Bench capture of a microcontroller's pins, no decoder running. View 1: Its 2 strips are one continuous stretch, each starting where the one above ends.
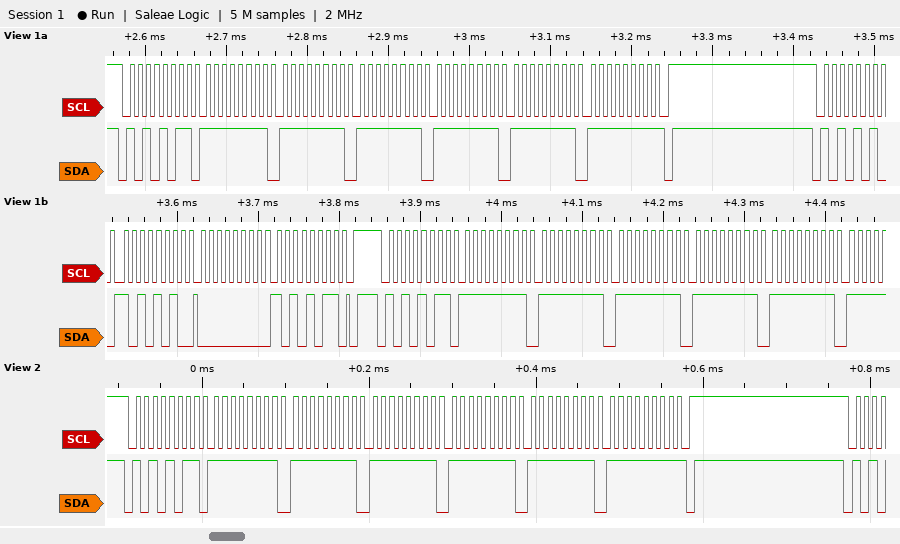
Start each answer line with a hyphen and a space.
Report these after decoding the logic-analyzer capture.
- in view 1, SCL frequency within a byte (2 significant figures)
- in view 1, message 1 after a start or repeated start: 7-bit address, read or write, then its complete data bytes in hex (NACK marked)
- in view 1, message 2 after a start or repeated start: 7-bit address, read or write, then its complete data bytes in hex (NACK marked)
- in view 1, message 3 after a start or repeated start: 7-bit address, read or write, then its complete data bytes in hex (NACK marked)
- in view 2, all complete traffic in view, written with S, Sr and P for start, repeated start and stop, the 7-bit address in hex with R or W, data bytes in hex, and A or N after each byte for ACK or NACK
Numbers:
- 100 kHz
- 0x55 read: FF FF FF FF FF FF NACK
- 0x55 write: AA 00 AB
- 0x55 read: FF FF FF FF FF
- S 55R A FF A FF A FF A FF A FF A FF N P
